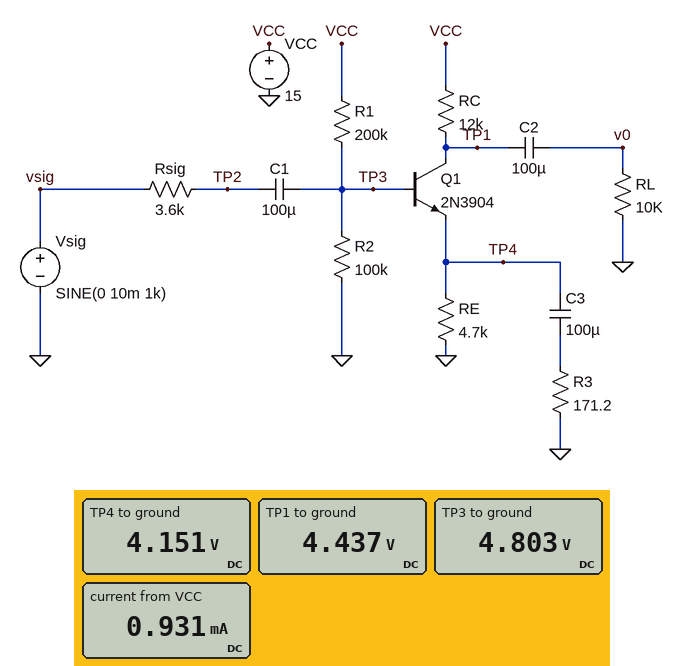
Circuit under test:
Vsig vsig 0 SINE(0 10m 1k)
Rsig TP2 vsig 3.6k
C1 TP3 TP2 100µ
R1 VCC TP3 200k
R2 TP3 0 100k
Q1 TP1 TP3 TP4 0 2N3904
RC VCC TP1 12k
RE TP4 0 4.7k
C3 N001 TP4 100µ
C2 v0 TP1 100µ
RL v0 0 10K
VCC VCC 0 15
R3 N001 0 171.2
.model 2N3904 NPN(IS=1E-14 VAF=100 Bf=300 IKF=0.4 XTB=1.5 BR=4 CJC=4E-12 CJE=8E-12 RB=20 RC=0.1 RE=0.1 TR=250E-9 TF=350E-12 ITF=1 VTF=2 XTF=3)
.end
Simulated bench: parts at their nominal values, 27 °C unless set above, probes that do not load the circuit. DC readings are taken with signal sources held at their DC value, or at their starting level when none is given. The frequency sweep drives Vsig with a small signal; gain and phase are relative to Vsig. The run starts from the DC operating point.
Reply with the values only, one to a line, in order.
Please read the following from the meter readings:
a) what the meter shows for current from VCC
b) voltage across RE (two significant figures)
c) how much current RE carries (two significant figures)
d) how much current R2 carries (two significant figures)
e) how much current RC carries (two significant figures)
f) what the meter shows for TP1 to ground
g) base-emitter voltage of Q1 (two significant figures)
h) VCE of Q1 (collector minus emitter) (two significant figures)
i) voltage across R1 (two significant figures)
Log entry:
0.931 mA
4.2 V
880 µA
48 µA
880 µA
4.437 V
650 mV
290 mV
10 V
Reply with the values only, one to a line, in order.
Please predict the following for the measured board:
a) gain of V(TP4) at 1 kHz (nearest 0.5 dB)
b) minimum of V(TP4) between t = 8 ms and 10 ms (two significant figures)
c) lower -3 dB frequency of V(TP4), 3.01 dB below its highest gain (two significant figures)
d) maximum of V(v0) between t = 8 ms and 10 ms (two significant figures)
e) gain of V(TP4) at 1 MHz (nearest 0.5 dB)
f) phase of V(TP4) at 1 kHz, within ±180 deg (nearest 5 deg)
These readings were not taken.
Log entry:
-2.5 dB
4.1 V
24 mHz
240 mV
-13.0 dB
0 deg
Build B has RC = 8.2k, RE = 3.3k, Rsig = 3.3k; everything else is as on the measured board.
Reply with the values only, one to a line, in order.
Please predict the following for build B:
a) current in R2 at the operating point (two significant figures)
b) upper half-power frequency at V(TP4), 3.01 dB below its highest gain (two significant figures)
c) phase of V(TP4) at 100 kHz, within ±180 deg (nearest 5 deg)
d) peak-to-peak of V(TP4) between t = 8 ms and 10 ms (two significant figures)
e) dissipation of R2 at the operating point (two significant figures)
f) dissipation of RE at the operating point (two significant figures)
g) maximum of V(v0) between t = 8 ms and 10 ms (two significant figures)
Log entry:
47 µA
340 kHz
-10 deg
16 mV
220 µW
5.0 mW
220 mV
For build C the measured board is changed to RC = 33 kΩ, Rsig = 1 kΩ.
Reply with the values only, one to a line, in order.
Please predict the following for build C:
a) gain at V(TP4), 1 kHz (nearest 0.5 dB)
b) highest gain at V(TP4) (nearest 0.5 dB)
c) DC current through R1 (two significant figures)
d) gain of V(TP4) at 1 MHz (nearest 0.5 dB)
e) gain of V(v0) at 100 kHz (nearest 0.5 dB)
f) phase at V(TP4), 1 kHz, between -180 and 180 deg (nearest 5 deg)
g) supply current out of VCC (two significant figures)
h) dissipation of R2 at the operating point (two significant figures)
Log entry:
-18.5 dB
-7.5 dB
62 µA
-17.5 dB
-12.5 dB
0 deg
450 µA
70 µW
